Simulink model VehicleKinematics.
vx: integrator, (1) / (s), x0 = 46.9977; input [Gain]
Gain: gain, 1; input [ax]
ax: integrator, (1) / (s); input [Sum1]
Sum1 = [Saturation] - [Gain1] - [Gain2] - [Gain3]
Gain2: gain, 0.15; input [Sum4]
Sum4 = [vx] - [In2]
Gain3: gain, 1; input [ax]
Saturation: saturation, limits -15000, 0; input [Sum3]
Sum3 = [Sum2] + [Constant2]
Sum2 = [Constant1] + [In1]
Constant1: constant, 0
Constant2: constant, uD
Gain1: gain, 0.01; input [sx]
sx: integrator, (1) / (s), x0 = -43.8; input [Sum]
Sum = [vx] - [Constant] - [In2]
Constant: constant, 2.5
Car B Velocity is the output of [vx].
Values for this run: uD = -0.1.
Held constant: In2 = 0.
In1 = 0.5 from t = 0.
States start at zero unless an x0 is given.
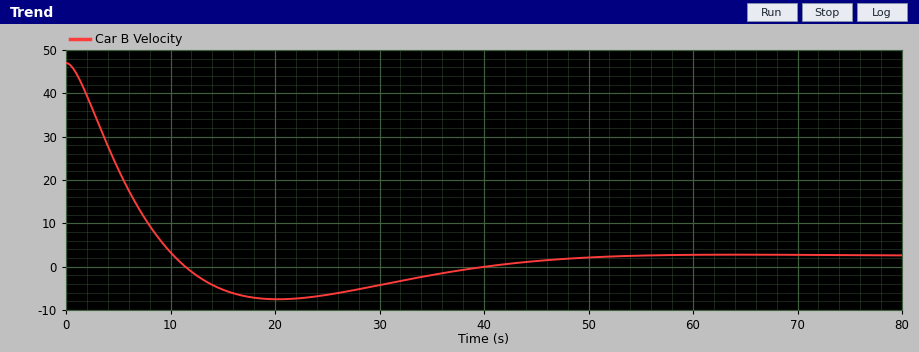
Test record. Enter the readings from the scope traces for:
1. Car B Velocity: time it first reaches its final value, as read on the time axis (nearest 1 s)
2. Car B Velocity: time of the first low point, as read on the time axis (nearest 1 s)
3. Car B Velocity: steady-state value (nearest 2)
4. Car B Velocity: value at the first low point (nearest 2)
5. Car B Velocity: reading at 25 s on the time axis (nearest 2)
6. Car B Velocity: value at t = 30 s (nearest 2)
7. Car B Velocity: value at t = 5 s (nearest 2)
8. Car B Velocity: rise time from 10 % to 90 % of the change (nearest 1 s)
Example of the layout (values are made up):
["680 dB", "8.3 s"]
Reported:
["10 s", "20 s", "2", "-8", "-6", "-4", "22", "7 s"]
